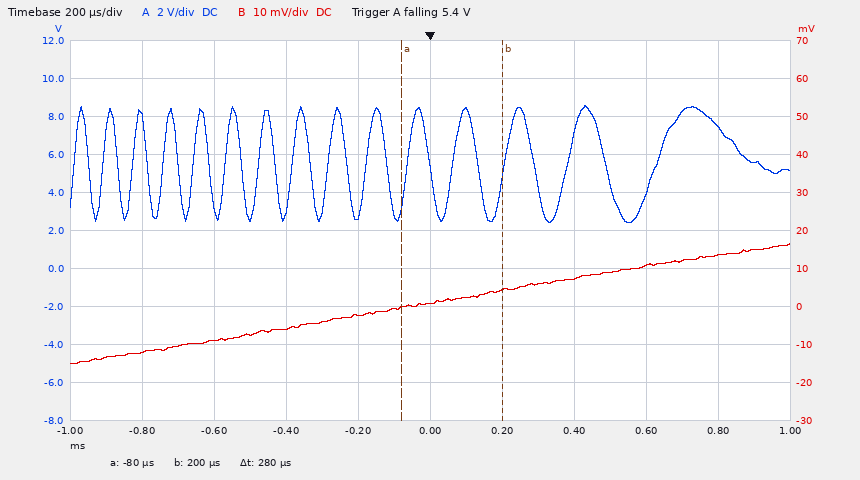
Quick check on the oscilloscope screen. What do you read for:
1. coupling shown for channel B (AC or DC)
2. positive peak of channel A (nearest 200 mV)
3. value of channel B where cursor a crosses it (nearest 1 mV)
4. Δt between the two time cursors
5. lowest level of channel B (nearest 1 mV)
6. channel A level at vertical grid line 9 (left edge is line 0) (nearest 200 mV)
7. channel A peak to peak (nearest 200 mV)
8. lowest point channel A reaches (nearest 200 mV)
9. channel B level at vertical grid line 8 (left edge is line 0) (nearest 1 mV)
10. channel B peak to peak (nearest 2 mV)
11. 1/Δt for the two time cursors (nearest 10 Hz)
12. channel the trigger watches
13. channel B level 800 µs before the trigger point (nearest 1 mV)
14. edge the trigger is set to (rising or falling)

DC
8.6 V
0 mV
280 µs
-15 mV
7.4 V
6.2 V
2.4 V
11 mV
32 mV
3.57 kHz
channel A
-12 mV
falling
